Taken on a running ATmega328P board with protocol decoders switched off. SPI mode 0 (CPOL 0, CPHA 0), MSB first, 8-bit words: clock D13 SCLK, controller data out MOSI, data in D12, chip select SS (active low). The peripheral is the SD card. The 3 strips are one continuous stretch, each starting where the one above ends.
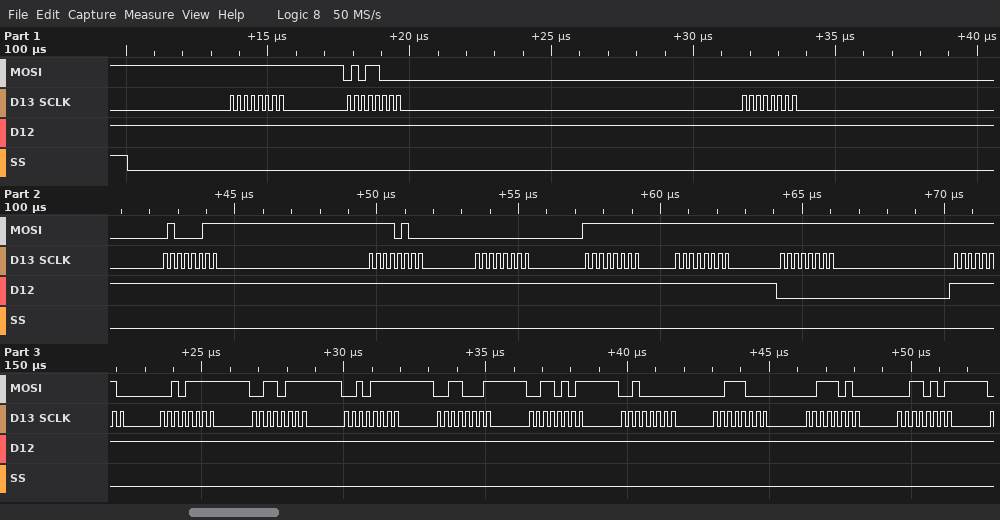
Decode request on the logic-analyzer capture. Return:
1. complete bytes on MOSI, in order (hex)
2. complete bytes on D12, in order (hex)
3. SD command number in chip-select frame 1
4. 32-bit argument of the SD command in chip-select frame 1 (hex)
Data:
0xFF 0x58 0x00 0x43 0xF4 0x00 0xFF 0xFF 0xFF 0xFE 0x2F 0x37 0x2F 0x31 0x35 0x20 0x38 0x3A 0x35
0xFF 0xFF 0xFF 0xFF 0xFF 0xFF 0xFF 0xFF 0x00 0xFF 0xFF 0xFF 0xFF 0xFF 0xFF 0xFF 0xFF 0xFF 0xFF
CMD24
0x0043F400
